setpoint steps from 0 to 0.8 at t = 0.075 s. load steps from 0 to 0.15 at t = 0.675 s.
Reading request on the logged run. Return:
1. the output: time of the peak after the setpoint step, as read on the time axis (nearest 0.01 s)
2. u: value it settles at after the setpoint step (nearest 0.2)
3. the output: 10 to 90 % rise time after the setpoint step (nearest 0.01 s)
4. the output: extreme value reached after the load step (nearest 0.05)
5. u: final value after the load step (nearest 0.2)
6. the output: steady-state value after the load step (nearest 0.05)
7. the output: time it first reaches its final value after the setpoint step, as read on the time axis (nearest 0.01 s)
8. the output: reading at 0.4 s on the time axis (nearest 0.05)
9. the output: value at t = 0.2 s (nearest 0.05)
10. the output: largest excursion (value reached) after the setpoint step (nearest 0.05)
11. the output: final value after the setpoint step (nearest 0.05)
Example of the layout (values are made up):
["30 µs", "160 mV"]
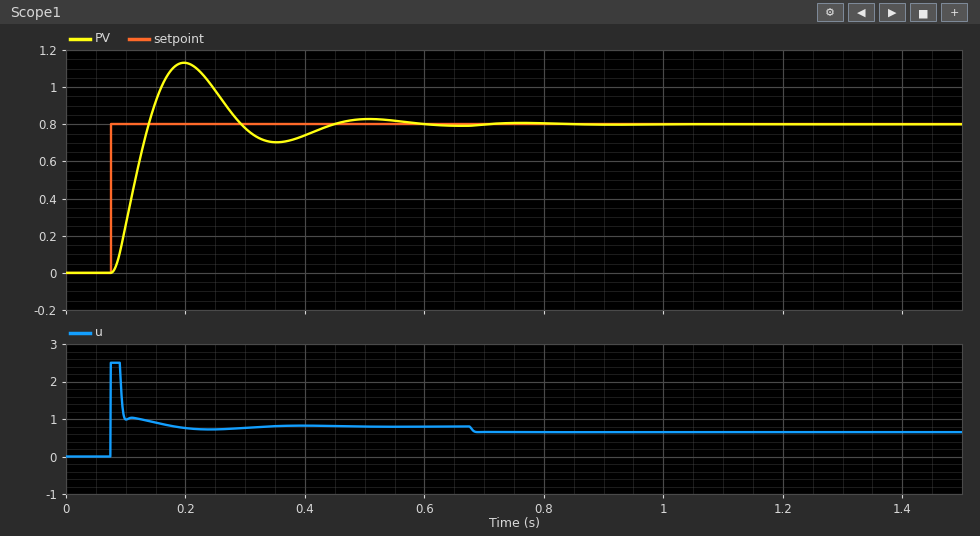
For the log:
["0.20 s", "0.8", "0.04 s", "0.80", "0.6", "0.80", "0.14 s", "0.75", "1.15", "1.15", "0.80"]
